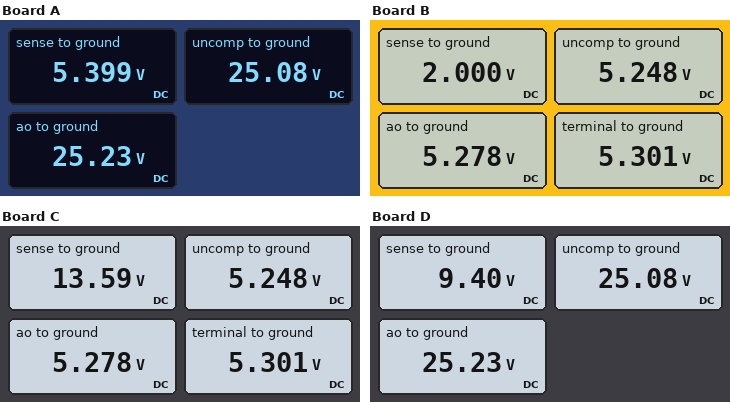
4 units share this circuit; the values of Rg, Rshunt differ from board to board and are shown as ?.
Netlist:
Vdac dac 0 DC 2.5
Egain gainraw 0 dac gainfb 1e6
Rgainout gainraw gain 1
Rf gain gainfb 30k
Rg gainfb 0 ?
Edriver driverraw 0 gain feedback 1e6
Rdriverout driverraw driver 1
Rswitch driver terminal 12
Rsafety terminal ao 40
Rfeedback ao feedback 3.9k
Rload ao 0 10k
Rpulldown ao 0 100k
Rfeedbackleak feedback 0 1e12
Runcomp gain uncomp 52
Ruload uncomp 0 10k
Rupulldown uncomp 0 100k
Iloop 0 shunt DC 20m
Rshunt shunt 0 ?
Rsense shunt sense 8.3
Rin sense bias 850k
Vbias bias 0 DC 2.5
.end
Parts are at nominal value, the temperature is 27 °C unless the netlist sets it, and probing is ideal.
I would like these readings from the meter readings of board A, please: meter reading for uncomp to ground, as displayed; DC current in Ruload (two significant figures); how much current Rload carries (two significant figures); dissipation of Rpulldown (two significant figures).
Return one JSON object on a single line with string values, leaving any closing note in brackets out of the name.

{"meter reading for uncomp to ground, as displayed": "25.08 V", "DC current in Ruload": "2.5 mA", "how much current Rload carries": "2.5 mA", "dissipation of Rpulldown": "6.4 mW"}
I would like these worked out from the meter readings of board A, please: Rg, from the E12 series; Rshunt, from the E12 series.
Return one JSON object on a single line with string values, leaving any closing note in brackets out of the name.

{"Rg, from the E12 series": "3.3 kΩ", "Rshunt, from the E12 series": "270 Ω"}
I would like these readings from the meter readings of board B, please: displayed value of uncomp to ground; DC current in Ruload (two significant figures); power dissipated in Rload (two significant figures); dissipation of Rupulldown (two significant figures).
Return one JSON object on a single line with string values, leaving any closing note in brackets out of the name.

{"displayed value of uncomp to ground": "5.248 V", "DC current in Ruload": "520 µA", "power dissipated in Rload": "2.8 mW", "dissipation of Rupulldown": "280 µW"}
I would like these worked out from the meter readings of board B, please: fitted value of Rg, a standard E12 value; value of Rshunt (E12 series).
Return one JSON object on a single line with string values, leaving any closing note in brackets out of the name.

{"fitted value of Rg, a standard E12 value": "27 kΩ", "value of Rshunt": "100 Ω"}
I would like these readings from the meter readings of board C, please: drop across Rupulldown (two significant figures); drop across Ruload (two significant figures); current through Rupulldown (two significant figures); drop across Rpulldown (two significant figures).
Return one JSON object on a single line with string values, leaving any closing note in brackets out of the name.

{"drop across Rupulldown": "5.2 V", "drop across Ruload": "5.2 V", "current through Rupulldown": "52 µA", "drop across Rpulldown": "5.3 V"}
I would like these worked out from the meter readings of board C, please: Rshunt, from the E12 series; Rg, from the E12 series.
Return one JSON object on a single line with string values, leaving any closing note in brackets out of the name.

{"Rshunt, from the E12 series": "680 Ω", "Rg, from the E12 series": "27 kΩ"}
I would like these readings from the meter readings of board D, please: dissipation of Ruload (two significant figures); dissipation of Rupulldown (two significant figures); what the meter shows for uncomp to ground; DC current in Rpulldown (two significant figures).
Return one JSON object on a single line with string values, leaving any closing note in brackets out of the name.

{"dissipation of Ruload": "63 mW", "dissipation of Rupulldown": "6.3 mW", "what the meter shows for uncomp to ground": "25.08 V", "DC current in Rpulldown": "250 µA"}
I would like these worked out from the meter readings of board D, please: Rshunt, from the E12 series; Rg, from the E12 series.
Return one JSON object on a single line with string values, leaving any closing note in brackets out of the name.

{"Rshunt, from the E12 series": "470 Ω", "Rg, from the E12 series": "3.3 kΩ"}
